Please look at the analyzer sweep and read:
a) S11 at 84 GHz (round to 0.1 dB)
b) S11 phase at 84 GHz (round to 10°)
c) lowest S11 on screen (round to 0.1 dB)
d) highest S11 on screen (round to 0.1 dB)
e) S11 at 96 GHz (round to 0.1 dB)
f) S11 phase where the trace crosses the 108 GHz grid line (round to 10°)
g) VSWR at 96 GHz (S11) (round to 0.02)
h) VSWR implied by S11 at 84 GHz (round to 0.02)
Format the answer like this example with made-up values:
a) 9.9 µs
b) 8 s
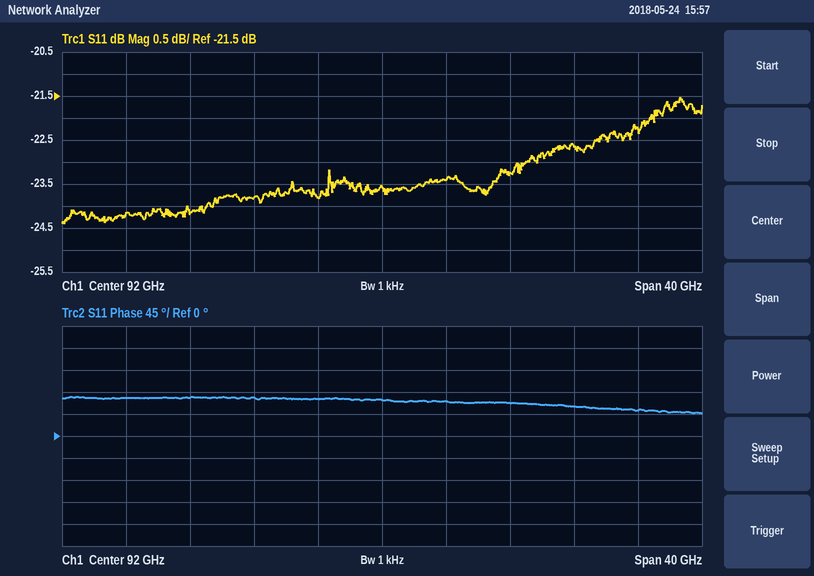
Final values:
a) -23.8 dB
b) 80°
c) -24.4 dB
d) -21.5 dB
e) -23.4 dB
f) 50°
g) 1.14
h) 1.14
